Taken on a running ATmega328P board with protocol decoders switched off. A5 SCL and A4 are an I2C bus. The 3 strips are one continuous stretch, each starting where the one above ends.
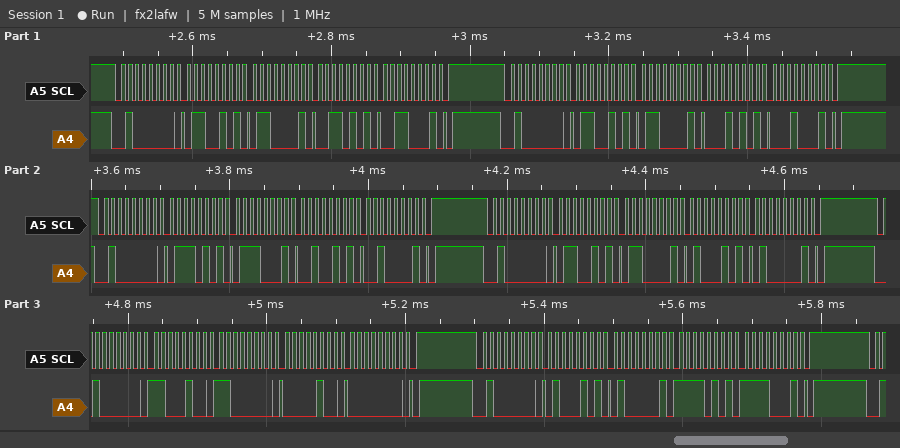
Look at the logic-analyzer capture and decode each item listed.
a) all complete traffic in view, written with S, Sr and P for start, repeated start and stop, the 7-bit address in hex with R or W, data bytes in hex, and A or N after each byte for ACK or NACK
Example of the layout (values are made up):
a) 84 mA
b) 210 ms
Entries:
a) S 20W A 65 A 61 A 35 A 31 A P S 20W A 65 A 61 A 15 A 11 A P S 20W A 75 A 71 A 25 A 21 A P S 20W A 65 A 61 A 45 A 41 A P S 20W A C4 A C0 A 04 A 00 A P S 20W A 45 A 41 A F5 A F1 A P
